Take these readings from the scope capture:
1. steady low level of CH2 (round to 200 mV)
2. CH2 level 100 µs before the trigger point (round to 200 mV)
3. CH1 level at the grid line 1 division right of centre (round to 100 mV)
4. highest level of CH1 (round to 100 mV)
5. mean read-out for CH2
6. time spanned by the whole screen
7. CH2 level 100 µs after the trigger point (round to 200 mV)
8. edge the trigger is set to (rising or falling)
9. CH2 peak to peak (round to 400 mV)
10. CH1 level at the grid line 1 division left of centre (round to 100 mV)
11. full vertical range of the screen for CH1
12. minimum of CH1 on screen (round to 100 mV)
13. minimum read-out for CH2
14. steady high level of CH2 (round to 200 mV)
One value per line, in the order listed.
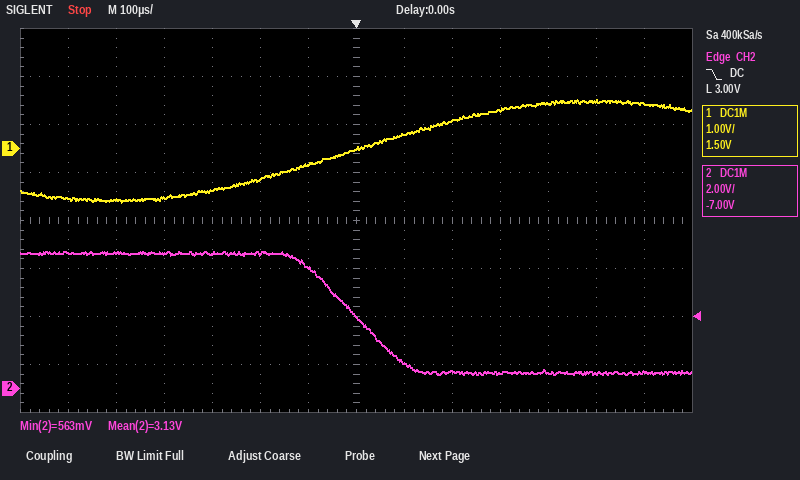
600 mV
5.0 V
300 mV
1.0 V
3.13 V
1.4 ms
1.0 V
falling
5.2 V
-300 mV
8 V
-1.1 V
563 mV
5.6 V
